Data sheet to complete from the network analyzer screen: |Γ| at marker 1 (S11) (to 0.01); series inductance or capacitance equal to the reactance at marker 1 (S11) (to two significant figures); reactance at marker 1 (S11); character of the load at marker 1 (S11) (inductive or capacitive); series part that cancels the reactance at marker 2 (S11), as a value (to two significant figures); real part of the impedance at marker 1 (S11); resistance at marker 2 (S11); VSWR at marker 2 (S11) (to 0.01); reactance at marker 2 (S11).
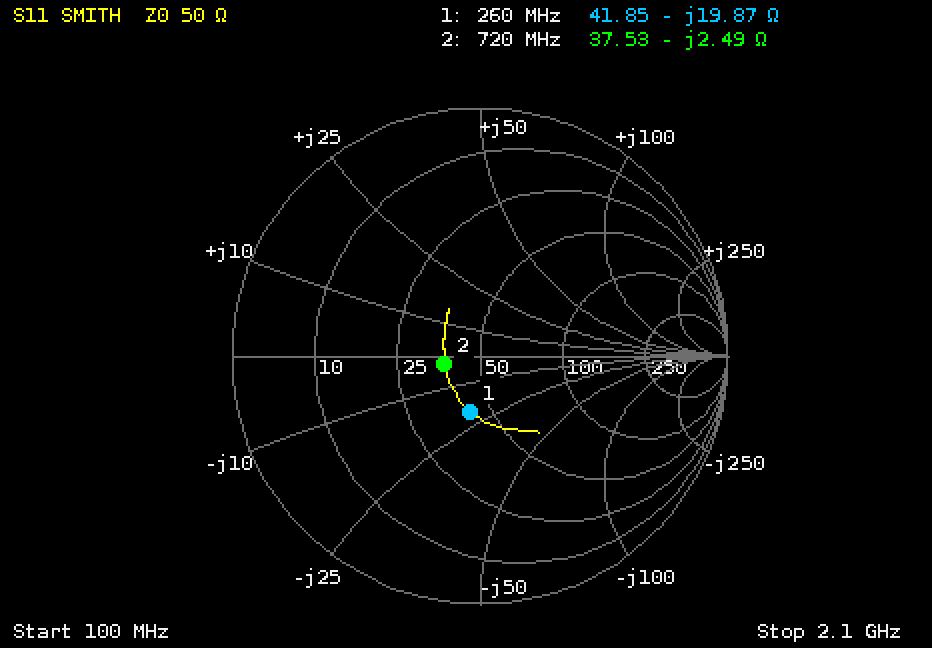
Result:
0.23
31 pF
-19.87 Ω
capacitive
550 pH
41.85 Ω
37.53 Ω
1.34
-2.49 Ω
